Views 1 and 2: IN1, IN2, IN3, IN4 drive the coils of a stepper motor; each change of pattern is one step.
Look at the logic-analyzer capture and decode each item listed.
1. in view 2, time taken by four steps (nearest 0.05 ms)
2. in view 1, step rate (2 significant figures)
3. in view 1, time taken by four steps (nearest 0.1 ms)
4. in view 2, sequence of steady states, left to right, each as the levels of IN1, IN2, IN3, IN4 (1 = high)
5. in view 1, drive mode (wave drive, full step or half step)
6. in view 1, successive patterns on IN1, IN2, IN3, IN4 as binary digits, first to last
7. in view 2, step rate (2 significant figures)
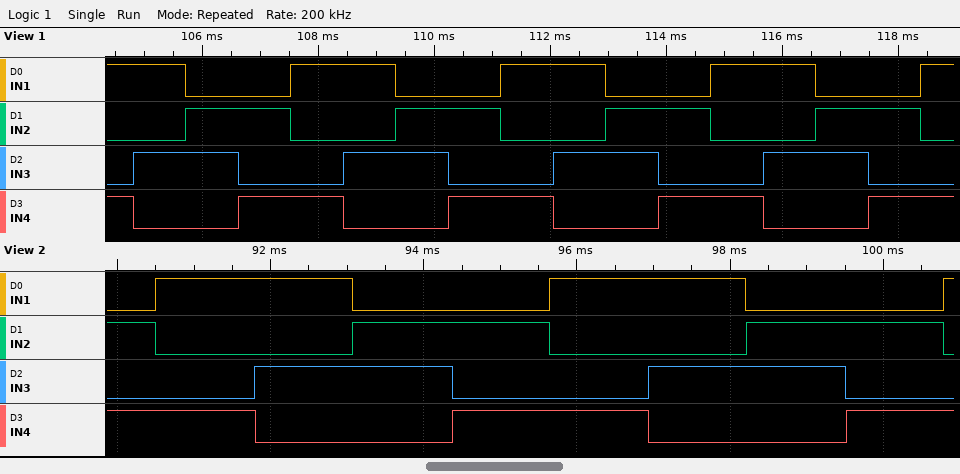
5.15 ms
1100 steps/s
3.6 ms
0101 1001 1010 0110 0101 1001 1010 0110 0101 1001
full step
1001 1010 0110 0101 1001 1010 0110 0101 1001 1010 0110 0101 1001 1010 0110 0101 1001
780 steps/s
